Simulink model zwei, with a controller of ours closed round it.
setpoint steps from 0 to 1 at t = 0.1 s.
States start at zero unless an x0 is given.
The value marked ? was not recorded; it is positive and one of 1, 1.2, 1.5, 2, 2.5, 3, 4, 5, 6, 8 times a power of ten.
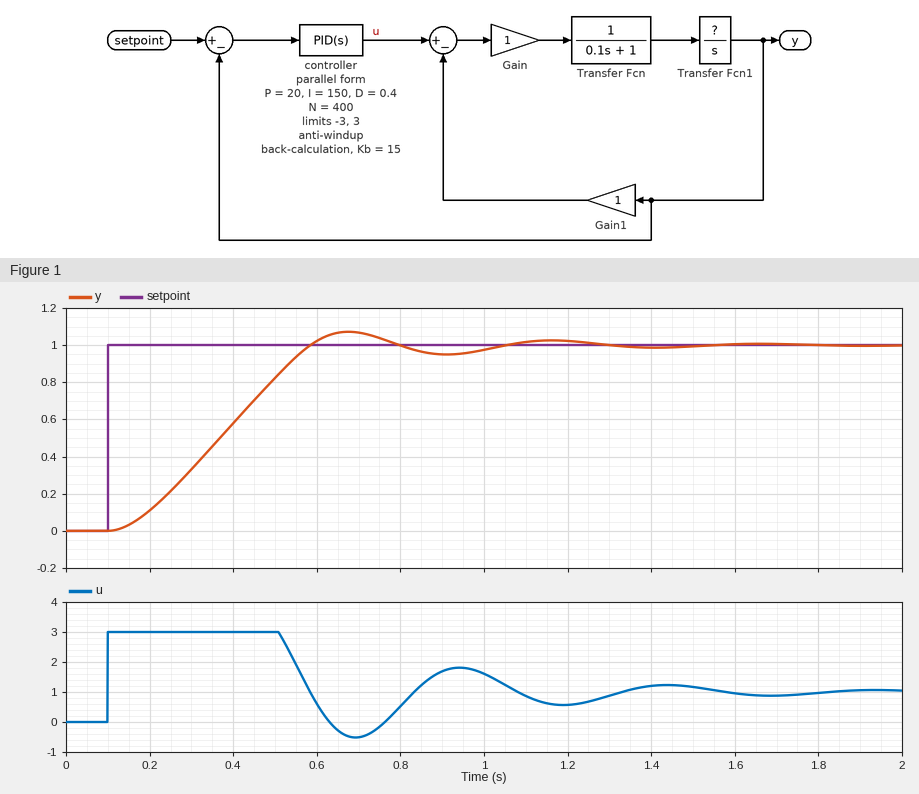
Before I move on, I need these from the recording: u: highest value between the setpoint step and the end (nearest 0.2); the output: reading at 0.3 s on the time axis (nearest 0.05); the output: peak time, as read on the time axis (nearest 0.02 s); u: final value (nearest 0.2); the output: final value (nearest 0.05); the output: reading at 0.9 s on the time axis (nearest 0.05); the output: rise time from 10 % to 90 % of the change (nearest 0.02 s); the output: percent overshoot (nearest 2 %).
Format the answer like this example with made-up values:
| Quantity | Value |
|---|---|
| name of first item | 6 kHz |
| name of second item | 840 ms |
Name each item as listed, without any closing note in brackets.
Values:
| Quantity | Value |
|---|---|
| u: highest value between the setpoint step and the end | 3.0 |
| the output: reading at 0.3 s on the time axis | 0.35 |
| the output: peak time, as read on the time axis | 0.68 s |
| u: final value | 1.0 |
| the output: final value | 1.00 |
| the output: reading at 0.9 s on the time axis | 0.95 |
| the output: rise time from 10 % to 90 % of the change | 0.34 s |
| the output: percent overshoot | 8 % |
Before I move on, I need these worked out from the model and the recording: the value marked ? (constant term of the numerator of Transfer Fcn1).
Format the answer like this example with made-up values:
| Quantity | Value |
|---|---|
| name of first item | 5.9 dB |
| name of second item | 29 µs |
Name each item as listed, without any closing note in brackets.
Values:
| Quantity | Value |
|---|---|
| the value marked ? | 1 |
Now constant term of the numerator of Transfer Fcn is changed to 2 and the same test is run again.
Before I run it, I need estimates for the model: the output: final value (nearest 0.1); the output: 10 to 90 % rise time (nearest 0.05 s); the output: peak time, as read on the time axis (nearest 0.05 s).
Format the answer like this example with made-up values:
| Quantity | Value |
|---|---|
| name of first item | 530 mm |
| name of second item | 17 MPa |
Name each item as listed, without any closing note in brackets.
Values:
| Quantity | Value |
|---|---|
| the output: final value | 1.0 |
| the output: 10 to 90 % rise time | 0.20 s |
| the output: peak time, as read on the time axis | 0.45 s |
